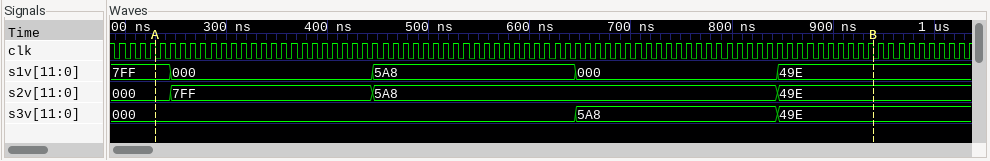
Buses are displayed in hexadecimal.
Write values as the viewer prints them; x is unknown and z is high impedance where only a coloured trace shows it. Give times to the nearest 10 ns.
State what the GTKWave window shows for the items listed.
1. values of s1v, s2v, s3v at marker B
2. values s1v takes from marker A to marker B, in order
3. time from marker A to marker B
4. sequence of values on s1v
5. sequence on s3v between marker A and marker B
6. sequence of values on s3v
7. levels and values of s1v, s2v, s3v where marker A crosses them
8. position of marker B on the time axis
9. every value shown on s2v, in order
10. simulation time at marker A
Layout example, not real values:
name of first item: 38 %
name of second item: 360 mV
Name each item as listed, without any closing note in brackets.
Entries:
values of s1v, s2v, s3v at marker B: s1v=49E, s2v=49E, s3v=49E
values s1v takes from marker A to marker B, in order: 7FF, 000, 5A8, 000, 49E
time from marker A to marker B: 710 ns
sequence of values on s1v: 7FF, 000, 5A8, 000, 49E
sequence on s3v between marker A and marker B: 000, 5A8, 49E
sequence of values on s3v: 000, 5A8, 49E
levels and values of s1v, s2v, s3v where marker A crosses them: s1v=7FF, s2v=000, s3v=000
position of marker B on the time axis: 940 ns
every value shown on s2v, in order: 000, 7FF, 5A8, 49E
simulation time at marker A: 230 ns
